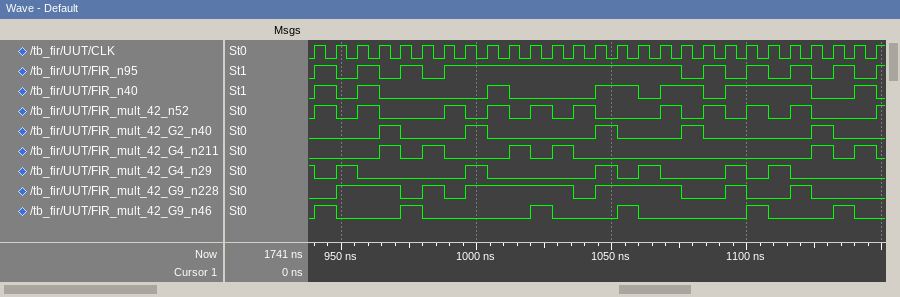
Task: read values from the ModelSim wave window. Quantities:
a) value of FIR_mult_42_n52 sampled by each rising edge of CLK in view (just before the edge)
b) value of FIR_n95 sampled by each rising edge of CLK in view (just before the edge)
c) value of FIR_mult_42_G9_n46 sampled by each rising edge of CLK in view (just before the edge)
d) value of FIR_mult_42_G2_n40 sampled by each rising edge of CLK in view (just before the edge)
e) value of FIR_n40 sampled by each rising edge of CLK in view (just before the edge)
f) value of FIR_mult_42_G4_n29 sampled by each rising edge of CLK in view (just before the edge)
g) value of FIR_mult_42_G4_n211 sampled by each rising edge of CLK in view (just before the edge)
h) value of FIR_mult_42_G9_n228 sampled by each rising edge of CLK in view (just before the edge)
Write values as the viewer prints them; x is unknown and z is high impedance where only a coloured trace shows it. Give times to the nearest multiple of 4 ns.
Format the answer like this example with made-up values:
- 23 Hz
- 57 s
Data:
- 0 1 0 1 0 0 0 1 0 1 0 1 0 1 0 0 0 1 0 1 0 1 0 1 0 0 0
- 0 1 0 1 0 1 0 1 1 1 1 1 1 1 1 1 1 1 0 1 0 1 0 1 0 1 0
- 0 1 0 0 0 1 0 0 0 0 0 1 0 0 0 1 0 0 0 0 0 1 0 0 0 1 0
- 0 0 0 0 1 0 0 0 1 0 0 0 0 0 1 0 0 0 1 0 0 0 0 0 1 0 0
- 0 1 0 1 0 0 0 0 0 1 0 0 0 0 1 1 0 1 1 0 1 1 1 1 0 0 1
- 1 0 1 0 0 0 0 0 1 0 0 0 0 0 1 0 1 0 0 0 1 0 1 0 0 0 0
- 0 0 0 0 1 0 1 0 0 0 1 0 1 0 0 0 0 0 0 0 0 0 0 0 1 0 1
- 0 0 1 1 1 0 1 0 1 1 1 1 1 0 1 1 1 1 0 0 1 0 0 1 0 0 0
